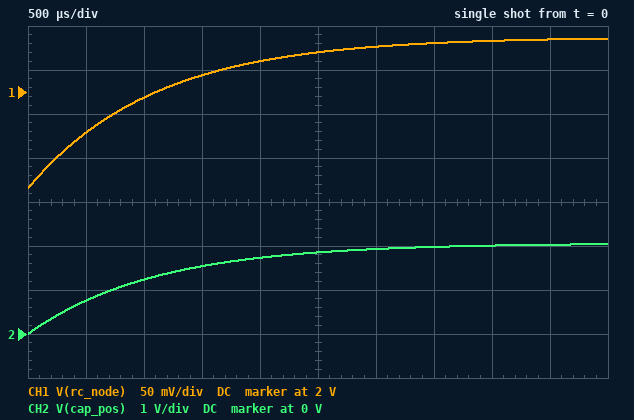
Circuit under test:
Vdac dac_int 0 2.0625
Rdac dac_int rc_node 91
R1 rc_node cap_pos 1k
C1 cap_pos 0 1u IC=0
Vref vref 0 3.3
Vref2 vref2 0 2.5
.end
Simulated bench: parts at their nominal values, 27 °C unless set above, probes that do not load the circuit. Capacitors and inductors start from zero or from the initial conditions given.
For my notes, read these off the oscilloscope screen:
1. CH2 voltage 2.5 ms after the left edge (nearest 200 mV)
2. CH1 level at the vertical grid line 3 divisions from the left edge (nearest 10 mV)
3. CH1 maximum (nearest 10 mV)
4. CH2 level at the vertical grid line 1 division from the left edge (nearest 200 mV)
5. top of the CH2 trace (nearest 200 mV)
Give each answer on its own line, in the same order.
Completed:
1.8 V
2.02 V
2.06 V
800 mV
2.0 V
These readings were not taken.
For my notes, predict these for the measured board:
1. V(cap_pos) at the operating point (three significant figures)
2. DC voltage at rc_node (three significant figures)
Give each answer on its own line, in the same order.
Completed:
2.06 V
2.06 V
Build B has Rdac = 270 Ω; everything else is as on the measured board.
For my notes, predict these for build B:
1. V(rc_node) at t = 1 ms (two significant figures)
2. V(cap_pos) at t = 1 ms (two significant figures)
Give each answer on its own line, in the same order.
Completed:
1.9 V
1.1 V
